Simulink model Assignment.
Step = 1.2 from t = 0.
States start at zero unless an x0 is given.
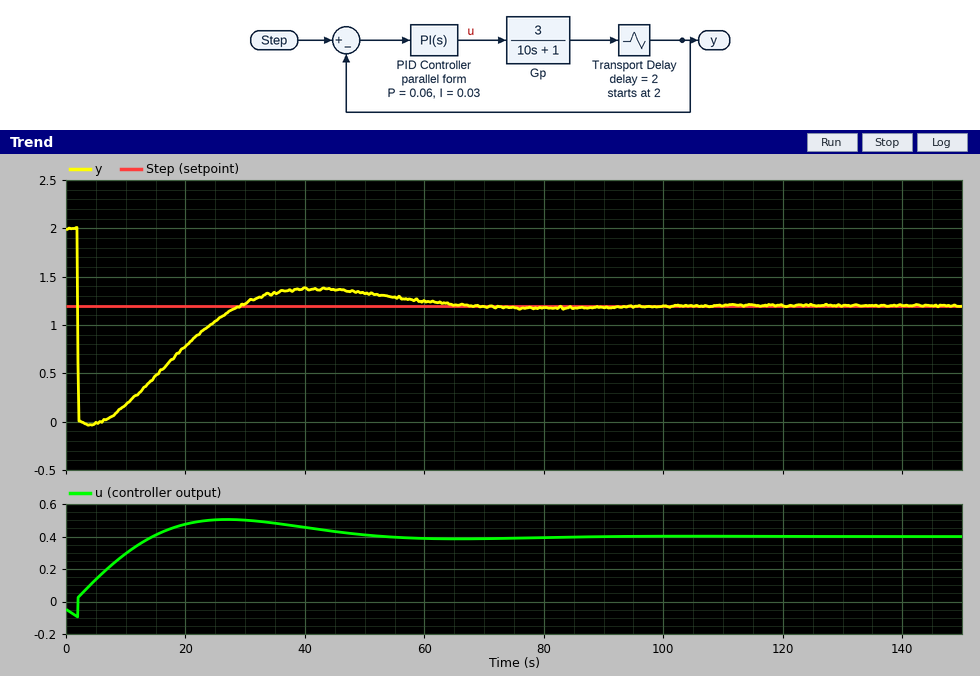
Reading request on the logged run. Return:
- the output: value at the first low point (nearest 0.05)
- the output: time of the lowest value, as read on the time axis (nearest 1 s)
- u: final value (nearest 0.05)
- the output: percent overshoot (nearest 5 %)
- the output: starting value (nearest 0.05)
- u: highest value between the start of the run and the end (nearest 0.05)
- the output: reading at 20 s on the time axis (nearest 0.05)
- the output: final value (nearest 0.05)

-0.05
4 s
0.40
155 %
2.00
0.50
0.80
1.20
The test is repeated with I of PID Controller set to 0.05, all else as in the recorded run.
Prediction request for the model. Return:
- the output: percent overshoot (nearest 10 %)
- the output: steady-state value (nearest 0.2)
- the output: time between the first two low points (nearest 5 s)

160 %
1.2
55 s
